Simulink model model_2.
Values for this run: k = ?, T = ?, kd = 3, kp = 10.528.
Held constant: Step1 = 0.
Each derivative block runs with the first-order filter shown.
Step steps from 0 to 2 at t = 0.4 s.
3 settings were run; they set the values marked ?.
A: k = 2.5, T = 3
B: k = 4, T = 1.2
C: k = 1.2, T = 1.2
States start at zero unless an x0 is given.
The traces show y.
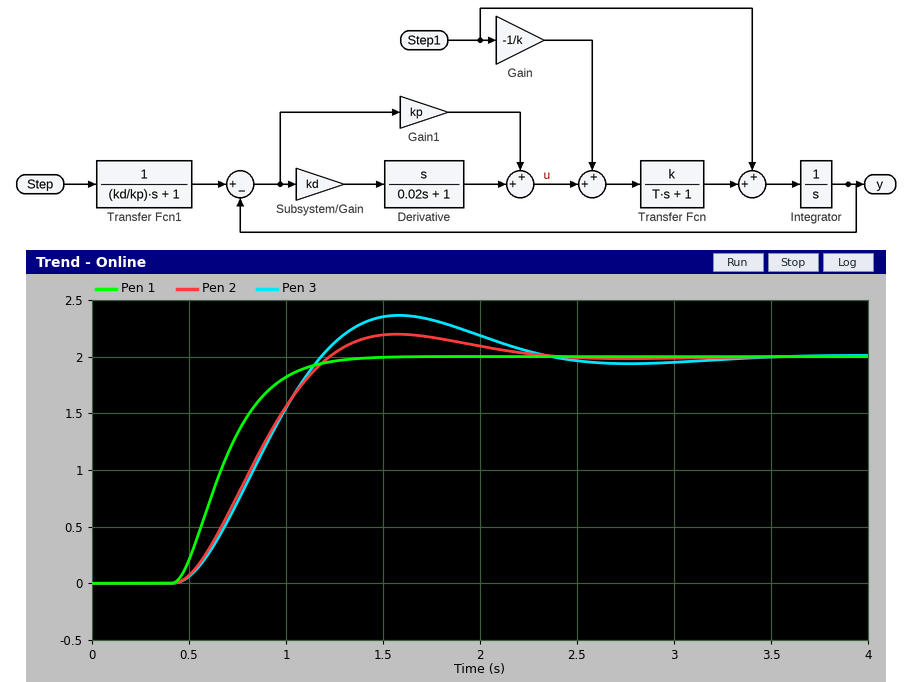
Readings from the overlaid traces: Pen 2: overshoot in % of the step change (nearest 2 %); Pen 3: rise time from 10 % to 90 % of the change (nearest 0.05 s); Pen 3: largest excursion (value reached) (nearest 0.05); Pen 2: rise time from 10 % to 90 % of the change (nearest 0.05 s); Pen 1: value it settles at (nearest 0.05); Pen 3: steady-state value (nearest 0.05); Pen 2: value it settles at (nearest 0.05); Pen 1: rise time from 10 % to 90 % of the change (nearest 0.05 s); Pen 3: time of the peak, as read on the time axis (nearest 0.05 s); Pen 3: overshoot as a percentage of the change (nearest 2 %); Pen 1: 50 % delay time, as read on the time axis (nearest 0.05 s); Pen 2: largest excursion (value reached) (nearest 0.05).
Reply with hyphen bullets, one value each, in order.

- 10 %
- 0.50 s
- 2.35
- 0.55 s
- 2.00
- 2.00
- 2.00
- 0.50 s
- 1.60 s
- 18 %
- 0.65 s
- 2.20
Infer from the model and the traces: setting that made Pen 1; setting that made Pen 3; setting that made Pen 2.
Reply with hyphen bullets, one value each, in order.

- B
- A
- C
